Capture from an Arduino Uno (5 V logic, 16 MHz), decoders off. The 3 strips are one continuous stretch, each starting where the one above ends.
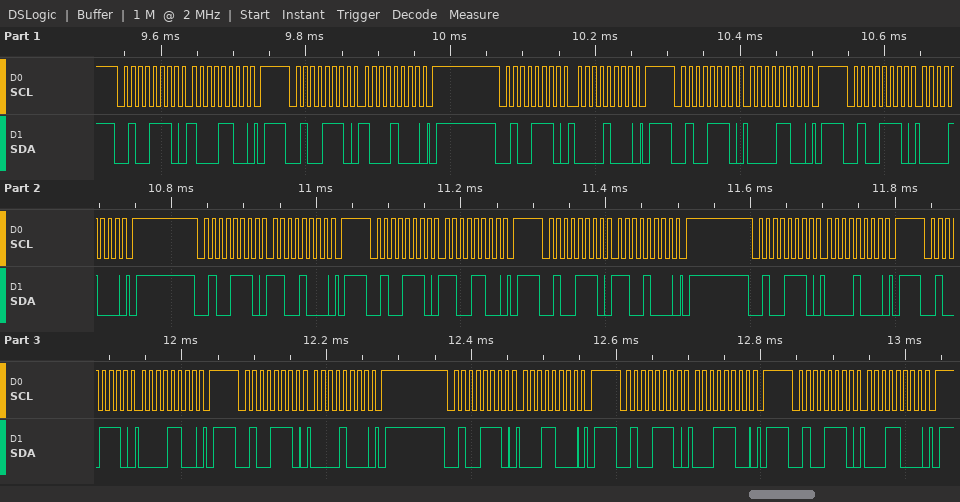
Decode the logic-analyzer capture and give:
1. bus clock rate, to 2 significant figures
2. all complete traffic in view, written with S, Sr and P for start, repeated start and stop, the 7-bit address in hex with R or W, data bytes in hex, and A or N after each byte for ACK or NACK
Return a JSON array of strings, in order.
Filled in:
["100 kHz", "S 27W A 8C A P S 27W A 88 A P S 27W A 08 A P S 27W A 0C A P S 27W A 08 A P S 27W A C8 A P S 27W A CC A P S 27W A C8 A P S 27W A 08 A P S 27W A 0C A P S 27W A 08 A P S 27W A 18 A P S 27W A 1C A P S 27W A 18 A P"]
